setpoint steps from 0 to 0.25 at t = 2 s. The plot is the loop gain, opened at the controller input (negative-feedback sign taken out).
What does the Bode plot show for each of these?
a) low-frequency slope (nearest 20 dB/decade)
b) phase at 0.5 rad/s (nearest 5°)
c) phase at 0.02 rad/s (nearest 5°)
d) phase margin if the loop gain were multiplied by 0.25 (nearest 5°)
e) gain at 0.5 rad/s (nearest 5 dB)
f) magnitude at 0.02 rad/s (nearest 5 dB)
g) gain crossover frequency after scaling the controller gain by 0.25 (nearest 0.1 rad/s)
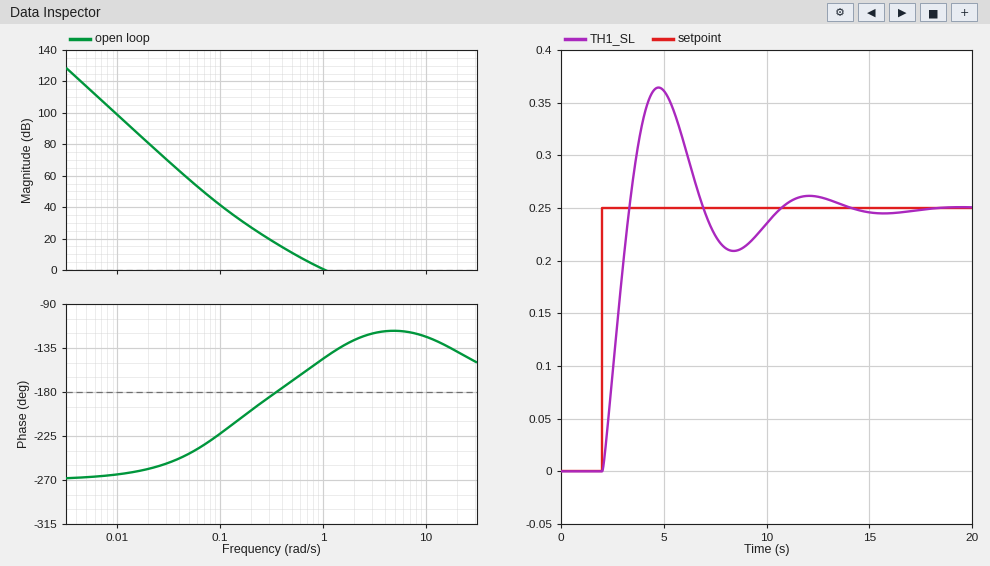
-60 dB/decade
-170°
-260°
10°
10 dB
80 dB
0.5 rad/s
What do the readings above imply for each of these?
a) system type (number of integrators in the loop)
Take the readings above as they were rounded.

3
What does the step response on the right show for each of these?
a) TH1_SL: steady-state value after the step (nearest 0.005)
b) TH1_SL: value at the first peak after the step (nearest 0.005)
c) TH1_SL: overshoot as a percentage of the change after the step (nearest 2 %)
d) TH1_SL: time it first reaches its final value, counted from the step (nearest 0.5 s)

0.250
0.365
46 %
1.5 s
